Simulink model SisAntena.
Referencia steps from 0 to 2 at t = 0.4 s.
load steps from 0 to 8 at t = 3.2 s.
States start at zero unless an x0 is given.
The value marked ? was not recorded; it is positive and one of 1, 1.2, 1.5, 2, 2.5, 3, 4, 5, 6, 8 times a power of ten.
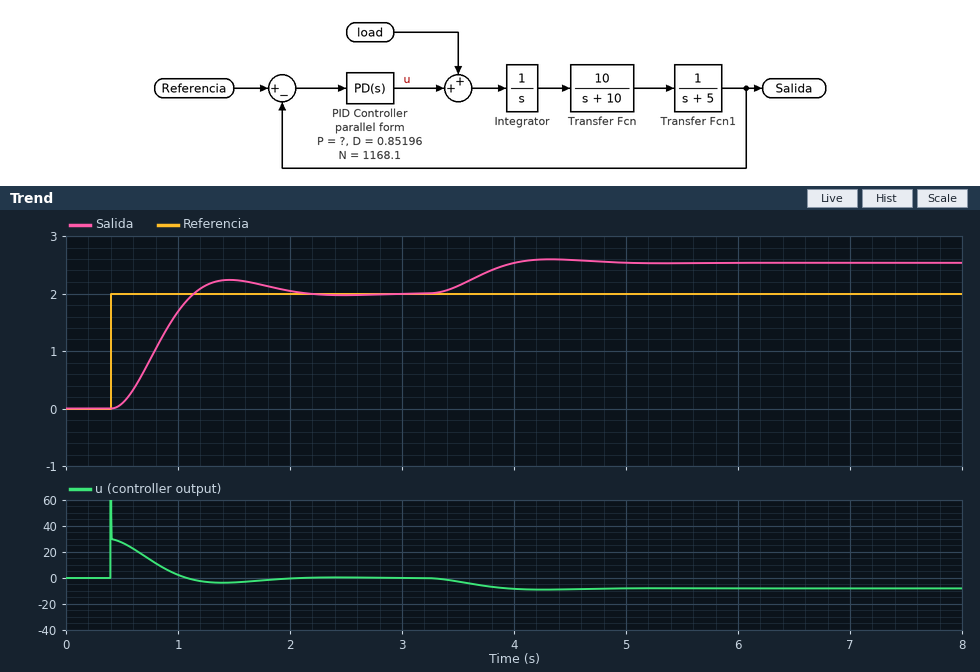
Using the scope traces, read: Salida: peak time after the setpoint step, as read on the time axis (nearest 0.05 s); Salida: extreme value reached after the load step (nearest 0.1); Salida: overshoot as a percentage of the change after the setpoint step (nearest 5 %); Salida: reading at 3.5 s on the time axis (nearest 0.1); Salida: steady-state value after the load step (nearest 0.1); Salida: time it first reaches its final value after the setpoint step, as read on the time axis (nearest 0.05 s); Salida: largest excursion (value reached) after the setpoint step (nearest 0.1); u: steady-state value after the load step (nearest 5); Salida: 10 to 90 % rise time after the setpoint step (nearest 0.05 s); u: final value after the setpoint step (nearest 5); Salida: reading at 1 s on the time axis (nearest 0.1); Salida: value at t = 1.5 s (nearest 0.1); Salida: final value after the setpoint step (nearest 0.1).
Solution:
1.45 s
2.6
10 %
2.1
2.5
1.15 s
2.2
-10
0.50 s
0
1.7
2.2
2.0
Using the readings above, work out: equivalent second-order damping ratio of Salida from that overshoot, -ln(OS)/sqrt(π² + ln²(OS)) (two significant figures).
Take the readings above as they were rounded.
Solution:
0.59
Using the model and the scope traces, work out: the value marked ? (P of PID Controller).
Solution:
15
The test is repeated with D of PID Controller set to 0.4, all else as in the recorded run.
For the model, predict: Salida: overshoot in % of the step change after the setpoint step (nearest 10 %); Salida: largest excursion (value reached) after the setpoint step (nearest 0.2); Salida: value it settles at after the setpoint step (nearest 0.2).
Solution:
20 %
2.4
2.0
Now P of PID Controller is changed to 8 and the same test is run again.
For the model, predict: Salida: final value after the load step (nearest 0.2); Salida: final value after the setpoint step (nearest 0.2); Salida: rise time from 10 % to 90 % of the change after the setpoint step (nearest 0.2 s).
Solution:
3.0
2.0
1.0 s
